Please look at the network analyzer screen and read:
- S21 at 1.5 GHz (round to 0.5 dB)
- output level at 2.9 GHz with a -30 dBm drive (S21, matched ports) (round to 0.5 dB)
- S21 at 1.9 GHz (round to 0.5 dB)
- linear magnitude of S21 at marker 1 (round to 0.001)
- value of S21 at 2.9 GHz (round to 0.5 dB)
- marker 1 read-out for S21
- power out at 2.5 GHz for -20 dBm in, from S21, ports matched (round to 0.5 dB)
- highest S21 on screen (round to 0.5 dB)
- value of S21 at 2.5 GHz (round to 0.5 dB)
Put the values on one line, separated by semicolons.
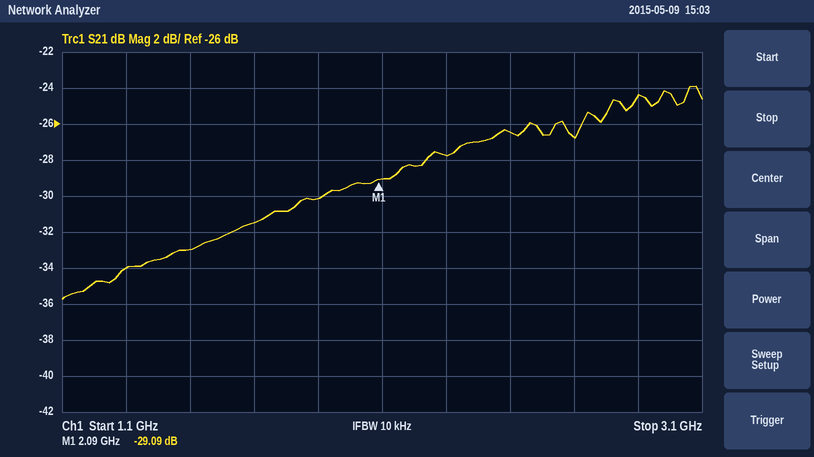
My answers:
-33.0 dB; -54.5 dBm; -30.0 dB; 0.035; -24.5 dB; -29.09 dB; -46.5 dBm; -24.0 dB; -26.5 dB
